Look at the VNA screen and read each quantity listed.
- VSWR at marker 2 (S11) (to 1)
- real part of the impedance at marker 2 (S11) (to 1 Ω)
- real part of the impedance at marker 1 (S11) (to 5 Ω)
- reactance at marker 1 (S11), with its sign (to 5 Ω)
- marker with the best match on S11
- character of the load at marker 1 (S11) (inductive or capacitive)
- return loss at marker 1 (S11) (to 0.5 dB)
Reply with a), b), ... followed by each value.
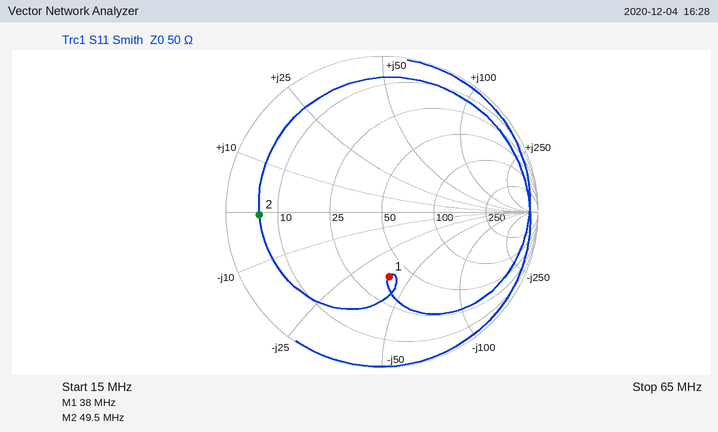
a) 8
b) 6 Ω
c) 40 Ω
d) -40 Ω
e) marker 1
f) capacitive
g) 7.5 dB
